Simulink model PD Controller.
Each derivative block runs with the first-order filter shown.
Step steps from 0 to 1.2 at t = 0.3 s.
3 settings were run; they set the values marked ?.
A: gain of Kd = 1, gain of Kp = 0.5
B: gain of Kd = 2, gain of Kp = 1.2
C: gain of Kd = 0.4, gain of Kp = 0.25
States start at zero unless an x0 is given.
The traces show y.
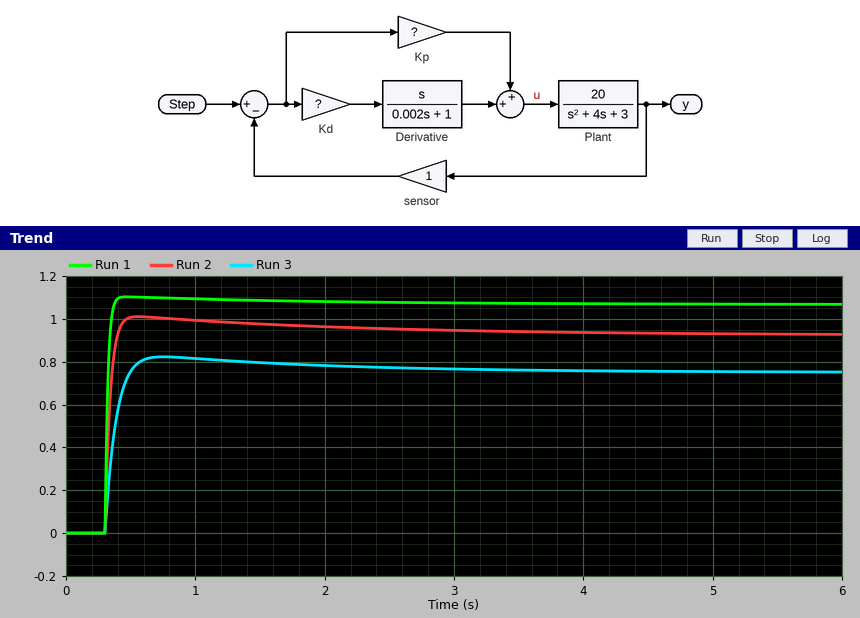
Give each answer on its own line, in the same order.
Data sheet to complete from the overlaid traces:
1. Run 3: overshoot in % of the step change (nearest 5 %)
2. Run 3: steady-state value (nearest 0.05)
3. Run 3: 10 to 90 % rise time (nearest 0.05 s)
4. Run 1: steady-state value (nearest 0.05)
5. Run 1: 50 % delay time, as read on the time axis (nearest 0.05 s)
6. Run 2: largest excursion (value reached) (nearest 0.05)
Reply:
10 %
0.75
0.15 s
1.05
0.30 s
1.00
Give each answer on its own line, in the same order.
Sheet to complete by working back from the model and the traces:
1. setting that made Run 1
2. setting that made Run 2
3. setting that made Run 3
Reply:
B
A
C
